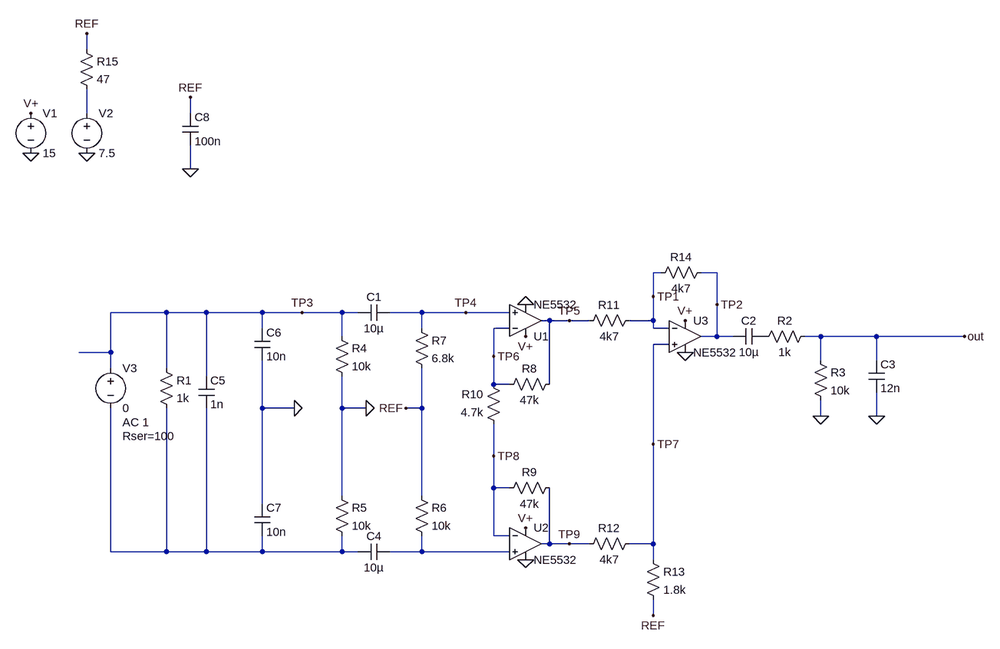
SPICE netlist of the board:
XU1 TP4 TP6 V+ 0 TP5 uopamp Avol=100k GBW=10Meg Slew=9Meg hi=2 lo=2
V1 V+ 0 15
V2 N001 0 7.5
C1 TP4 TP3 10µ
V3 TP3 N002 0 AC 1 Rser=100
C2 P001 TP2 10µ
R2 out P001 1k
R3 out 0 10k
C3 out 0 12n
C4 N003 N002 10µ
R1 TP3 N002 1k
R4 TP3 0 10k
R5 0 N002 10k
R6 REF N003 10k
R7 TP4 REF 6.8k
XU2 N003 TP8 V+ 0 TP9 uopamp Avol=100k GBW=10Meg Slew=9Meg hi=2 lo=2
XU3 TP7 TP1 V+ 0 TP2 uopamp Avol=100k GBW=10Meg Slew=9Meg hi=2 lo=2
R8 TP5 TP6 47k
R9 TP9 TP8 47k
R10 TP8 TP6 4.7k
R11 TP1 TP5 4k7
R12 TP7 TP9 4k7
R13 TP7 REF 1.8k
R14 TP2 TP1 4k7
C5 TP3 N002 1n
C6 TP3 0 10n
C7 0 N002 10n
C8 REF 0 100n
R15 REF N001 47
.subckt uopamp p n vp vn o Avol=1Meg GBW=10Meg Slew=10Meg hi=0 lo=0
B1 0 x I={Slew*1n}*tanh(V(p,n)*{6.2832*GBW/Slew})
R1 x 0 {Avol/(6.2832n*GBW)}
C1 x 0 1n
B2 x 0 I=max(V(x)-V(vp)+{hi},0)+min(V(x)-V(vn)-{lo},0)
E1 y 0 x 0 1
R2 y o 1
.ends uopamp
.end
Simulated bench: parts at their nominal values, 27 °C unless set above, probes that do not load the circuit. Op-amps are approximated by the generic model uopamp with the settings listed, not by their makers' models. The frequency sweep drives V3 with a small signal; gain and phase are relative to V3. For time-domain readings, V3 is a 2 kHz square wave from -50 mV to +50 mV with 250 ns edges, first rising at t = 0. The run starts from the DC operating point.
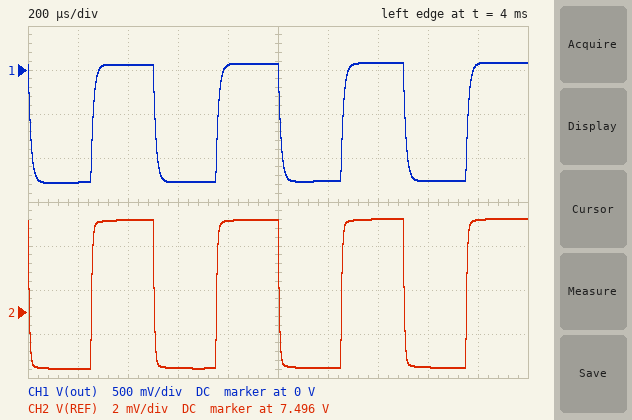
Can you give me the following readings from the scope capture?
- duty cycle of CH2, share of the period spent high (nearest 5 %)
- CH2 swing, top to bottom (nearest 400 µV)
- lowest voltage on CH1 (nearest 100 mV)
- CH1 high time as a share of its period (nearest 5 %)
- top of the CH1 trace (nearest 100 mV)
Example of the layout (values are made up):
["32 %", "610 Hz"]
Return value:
["50 %", "6.8 mV", "-1.3 V", "50 %", "100 mV"]
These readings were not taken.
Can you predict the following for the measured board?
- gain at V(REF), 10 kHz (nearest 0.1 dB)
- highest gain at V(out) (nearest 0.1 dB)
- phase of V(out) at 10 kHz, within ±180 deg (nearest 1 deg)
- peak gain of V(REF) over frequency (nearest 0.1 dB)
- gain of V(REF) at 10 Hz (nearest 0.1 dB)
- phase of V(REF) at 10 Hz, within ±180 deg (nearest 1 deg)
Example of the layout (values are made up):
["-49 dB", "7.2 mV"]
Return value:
["-23.9 dB", "22.5 dB", "142 deg", "-23.4 dB", "-23.6 dB", "-169 deg"]
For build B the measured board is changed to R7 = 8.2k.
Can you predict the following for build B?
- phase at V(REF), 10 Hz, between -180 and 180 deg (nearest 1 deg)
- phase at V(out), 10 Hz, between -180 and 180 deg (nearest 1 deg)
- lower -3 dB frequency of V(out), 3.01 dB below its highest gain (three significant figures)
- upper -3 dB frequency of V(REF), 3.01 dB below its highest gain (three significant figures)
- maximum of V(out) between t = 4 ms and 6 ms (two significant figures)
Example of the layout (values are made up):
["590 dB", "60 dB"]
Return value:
["-170 deg", "-162 deg", "2.50 Hz", "32.8 kHz", "78 mV"]
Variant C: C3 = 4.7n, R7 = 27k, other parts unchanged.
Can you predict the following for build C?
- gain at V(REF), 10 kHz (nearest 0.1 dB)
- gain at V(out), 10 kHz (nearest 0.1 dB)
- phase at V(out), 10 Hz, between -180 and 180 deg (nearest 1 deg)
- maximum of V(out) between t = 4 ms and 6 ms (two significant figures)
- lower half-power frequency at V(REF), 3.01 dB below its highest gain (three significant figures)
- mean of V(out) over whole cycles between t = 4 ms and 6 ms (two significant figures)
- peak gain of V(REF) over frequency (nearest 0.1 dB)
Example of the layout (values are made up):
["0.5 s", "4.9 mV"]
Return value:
["-23.6 dB", "22.3 dB", "-166 deg", "59 mV", "980 mHz", "-620 mV", "-23.3 dB"]
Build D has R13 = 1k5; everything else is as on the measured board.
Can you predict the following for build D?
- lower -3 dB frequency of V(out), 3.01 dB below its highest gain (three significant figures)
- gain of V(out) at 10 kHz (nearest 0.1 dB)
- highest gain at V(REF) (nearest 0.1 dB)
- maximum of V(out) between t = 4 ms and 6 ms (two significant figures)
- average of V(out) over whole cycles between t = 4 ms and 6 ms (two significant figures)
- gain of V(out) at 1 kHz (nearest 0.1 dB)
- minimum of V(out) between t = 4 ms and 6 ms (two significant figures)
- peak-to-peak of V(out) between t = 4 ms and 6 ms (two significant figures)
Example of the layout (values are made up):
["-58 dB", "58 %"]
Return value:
["2.66 Hz", "20.5 dB", "-23.0 dB", "78 mV", "-570 mV", "22.1 dB", "-1.2 V", "1.3 V"]
